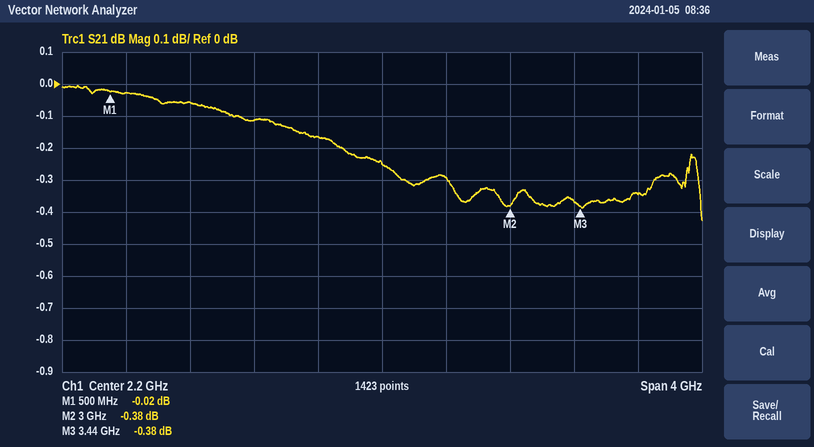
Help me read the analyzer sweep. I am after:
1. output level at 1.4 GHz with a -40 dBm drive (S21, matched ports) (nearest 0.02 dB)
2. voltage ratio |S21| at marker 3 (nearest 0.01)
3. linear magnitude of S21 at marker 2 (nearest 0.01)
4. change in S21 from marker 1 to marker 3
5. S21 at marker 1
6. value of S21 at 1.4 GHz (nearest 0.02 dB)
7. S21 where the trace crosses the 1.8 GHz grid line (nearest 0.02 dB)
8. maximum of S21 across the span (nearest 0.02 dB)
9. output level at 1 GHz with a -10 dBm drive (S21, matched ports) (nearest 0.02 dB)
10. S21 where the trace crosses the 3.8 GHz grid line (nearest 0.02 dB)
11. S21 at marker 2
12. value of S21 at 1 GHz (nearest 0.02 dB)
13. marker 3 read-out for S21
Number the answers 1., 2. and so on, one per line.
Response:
1. -40.12 dBm
2. 0.96
3. 0.96
4. -0.36 dB
5. -0.02 dB
6. -0.12 dB
7. -0.16 dB
8. 0.00 dB
9. -10.06 dBm
10. -0.34 dB
11. -0.38 dB
12. -0.06 dB
13. -0.38 dB
